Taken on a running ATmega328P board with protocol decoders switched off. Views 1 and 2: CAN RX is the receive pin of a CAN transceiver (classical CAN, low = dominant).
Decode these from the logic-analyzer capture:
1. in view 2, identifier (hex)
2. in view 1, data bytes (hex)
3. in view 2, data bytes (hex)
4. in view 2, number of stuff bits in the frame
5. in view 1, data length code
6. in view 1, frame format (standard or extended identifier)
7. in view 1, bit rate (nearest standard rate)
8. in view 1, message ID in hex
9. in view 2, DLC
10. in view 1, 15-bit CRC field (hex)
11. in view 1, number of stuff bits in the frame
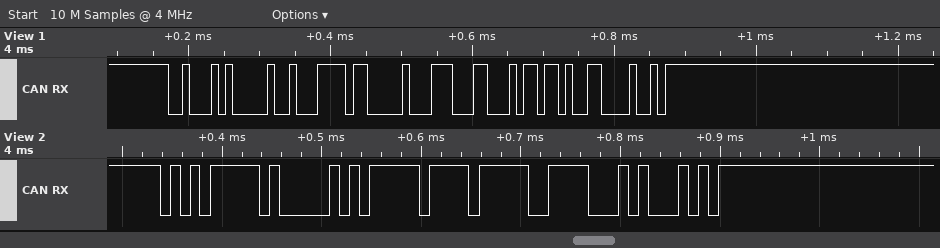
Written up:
0x57E
7B 00 E3 16
FF BE
4
4
standard
100 kbit/s
0x228
2
0x6984
2
